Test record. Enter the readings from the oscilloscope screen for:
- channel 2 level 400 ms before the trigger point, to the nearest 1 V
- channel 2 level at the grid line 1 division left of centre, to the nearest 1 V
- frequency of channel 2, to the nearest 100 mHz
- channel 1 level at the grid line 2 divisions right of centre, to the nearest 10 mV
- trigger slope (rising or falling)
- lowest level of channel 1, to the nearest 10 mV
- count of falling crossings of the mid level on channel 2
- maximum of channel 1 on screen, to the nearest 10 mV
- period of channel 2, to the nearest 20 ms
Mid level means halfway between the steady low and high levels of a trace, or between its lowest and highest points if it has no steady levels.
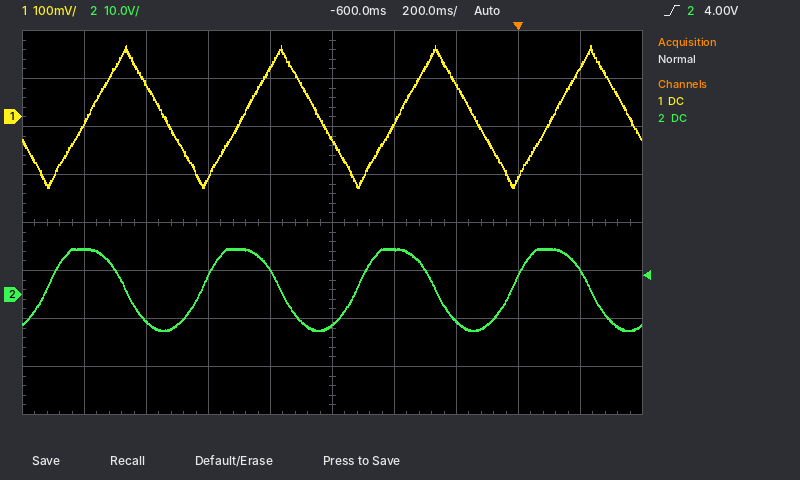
9 V
5 V
2.0 Hz
70 mV
rising
-150 mV
4
150 mV
500 ms
